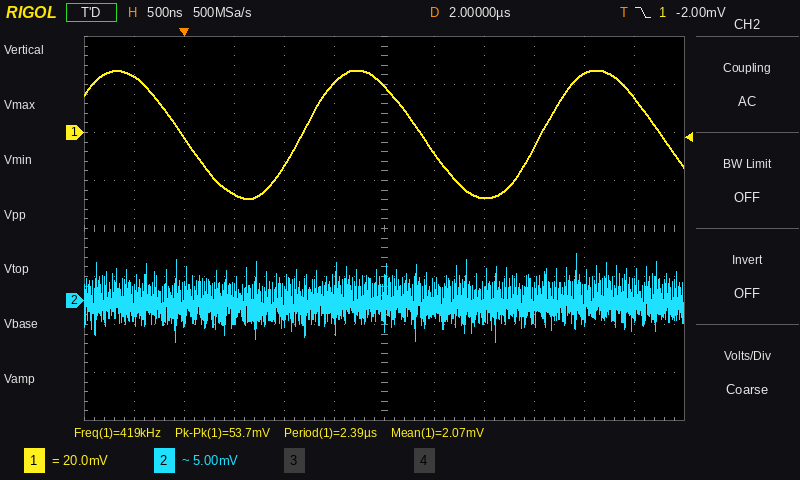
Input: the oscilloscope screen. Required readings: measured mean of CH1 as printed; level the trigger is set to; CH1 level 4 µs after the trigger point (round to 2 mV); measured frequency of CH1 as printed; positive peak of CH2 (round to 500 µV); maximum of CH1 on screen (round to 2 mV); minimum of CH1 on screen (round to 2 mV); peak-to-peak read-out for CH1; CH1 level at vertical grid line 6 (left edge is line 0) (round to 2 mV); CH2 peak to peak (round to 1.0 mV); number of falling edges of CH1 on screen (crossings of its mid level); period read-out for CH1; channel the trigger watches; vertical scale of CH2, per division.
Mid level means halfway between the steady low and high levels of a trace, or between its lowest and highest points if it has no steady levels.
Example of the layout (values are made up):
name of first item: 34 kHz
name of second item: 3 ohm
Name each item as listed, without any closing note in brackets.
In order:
measured mean of CH1 as printed: 2.07 mV
level the trigger is set to: -2.00 mV
CH1 level 4 µs after the trigger point: 24 mV
measured frequency of CH1 as printed: 419 kHz
positive peak of CH2: 5.0 mV
maximum of CH1 on screen: 26 mV
minimum of CH1 on screen: -28 mV
peak-to-peak read-out for CH1: 53.7 mV
CH1 level at vertical grid line 6 (left edge is line 0): 20 mV
CH2 peak to peak: 9.0 mV
number of falling edges of CH1 on screen: 3
period read-out for CH1: 2.39 µs
channel the trigger watches: CH1
vertical scale of CH2, per division: 5 mV
